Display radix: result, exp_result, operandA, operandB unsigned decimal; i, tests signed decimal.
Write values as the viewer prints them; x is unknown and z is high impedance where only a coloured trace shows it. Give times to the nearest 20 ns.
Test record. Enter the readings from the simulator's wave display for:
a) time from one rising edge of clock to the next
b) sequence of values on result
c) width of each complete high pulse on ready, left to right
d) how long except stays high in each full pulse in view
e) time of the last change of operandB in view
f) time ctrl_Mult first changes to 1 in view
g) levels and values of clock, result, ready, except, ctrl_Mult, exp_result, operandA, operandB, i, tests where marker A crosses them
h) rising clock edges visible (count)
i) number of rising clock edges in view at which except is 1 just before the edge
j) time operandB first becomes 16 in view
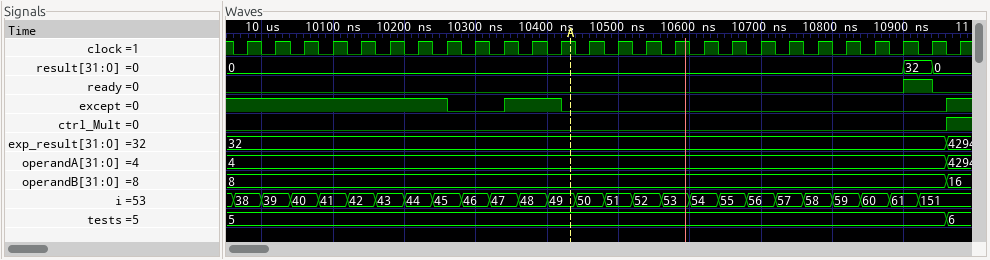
40 ns
0, 32, 0
40 ns
80 ns
10960 ns
10960 ns
clock=1, result=0, ready=0, except=0, ctrl_Mult=0, exp_result=32, operandA=4, operandB=8, i=49, tests=5
26
11
10960 ns
